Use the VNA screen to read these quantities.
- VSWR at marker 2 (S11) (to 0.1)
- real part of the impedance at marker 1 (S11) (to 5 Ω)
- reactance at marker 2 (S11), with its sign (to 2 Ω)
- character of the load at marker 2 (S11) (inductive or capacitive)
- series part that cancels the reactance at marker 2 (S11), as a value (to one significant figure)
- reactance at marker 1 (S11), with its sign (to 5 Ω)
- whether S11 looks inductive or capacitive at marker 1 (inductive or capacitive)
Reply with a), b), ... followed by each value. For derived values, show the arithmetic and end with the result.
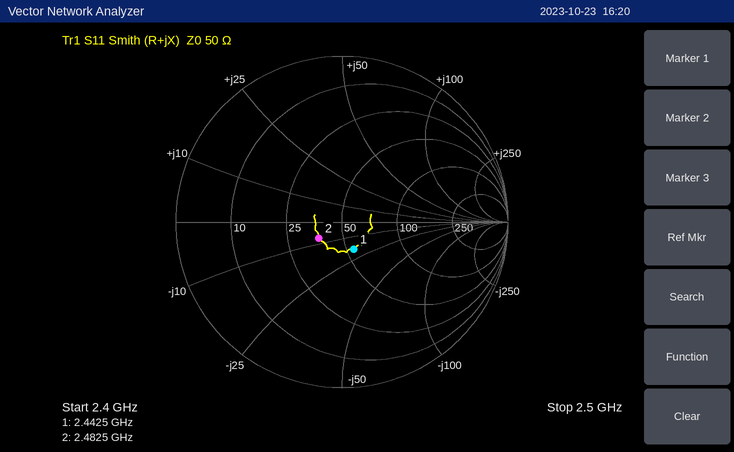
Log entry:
a) 1.4
b) 55 Ω
c) -8 Ω
d) capacitive
e) L = 8 Ω/(2π × 2.4825 GHz) ≈ 513 pH, so 500 pH to one significant figure
f) -20 Ω
g) capacitive
